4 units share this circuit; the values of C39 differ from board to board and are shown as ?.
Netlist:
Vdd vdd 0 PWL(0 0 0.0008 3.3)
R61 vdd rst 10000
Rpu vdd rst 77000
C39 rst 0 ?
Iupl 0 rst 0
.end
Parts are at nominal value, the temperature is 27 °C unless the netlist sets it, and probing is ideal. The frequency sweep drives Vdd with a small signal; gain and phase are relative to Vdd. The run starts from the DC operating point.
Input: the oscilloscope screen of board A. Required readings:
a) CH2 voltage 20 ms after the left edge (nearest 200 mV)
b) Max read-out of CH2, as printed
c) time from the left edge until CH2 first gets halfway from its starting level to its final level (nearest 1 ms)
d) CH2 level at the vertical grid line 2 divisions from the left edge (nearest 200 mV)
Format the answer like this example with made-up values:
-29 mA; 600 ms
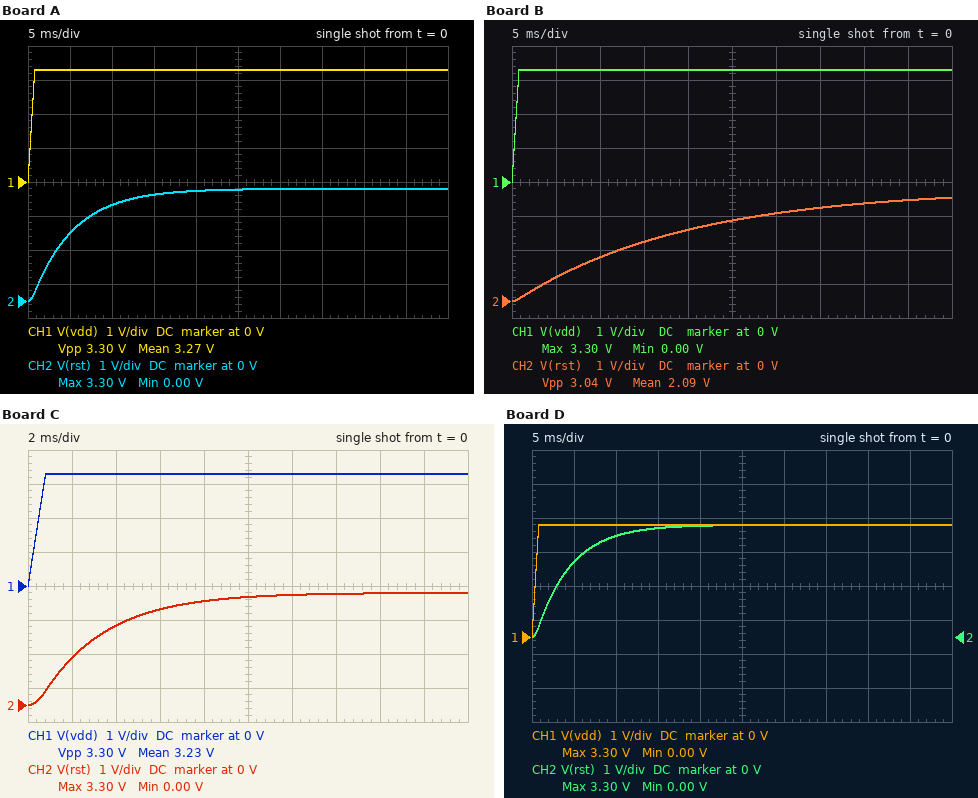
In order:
3.2 V; 3.30 V; 4 ms; 2.8 V
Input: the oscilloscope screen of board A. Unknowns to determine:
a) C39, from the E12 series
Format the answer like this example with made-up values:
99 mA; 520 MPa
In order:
560 nF
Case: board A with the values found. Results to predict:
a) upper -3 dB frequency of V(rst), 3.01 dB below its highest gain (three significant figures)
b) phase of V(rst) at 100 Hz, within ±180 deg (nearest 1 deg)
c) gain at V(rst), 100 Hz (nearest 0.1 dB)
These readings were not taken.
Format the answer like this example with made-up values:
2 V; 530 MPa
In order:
32.1 Hz; -72 deg; -10.3 dB
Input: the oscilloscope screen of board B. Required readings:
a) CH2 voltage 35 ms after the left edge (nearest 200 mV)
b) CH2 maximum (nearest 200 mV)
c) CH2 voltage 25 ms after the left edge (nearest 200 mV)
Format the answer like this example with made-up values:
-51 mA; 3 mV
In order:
2.8 V; 3.0 V; 2.4 V
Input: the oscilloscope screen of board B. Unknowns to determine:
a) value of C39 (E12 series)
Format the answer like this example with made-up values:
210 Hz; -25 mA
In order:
2.2 µF
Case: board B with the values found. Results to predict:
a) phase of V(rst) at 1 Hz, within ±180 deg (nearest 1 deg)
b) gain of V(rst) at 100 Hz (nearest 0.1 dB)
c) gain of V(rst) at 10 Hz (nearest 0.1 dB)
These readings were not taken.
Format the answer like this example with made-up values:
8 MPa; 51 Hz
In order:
-7 deg; -21.8 dB; -4.0 dB
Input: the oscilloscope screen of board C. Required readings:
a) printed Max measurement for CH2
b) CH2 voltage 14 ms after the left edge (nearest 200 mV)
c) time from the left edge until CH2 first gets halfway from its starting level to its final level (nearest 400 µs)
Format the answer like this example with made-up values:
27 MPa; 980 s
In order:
3.30 V; 3.2 V; 2.4 ms
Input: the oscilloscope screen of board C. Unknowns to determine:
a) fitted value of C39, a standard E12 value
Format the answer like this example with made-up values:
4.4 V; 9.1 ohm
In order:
330 nF
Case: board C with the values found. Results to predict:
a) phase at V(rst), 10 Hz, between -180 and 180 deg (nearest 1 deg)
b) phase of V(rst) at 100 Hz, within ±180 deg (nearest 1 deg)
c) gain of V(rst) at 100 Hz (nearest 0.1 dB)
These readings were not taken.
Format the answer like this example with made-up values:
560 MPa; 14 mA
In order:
-10 deg; -61 deg; -6.4 dB
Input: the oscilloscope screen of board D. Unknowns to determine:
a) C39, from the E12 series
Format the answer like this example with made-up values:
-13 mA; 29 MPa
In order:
470 nF
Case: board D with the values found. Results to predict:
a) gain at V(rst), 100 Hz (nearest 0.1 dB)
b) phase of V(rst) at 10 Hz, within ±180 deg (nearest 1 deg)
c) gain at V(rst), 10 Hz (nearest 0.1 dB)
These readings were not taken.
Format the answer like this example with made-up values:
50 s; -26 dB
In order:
-8.9 dB; -15 deg; -0.3 dB
